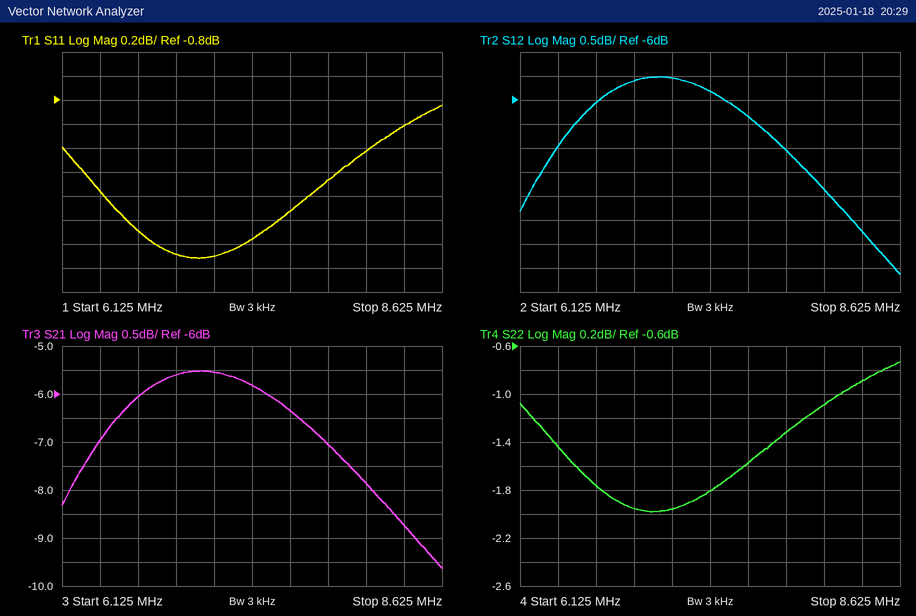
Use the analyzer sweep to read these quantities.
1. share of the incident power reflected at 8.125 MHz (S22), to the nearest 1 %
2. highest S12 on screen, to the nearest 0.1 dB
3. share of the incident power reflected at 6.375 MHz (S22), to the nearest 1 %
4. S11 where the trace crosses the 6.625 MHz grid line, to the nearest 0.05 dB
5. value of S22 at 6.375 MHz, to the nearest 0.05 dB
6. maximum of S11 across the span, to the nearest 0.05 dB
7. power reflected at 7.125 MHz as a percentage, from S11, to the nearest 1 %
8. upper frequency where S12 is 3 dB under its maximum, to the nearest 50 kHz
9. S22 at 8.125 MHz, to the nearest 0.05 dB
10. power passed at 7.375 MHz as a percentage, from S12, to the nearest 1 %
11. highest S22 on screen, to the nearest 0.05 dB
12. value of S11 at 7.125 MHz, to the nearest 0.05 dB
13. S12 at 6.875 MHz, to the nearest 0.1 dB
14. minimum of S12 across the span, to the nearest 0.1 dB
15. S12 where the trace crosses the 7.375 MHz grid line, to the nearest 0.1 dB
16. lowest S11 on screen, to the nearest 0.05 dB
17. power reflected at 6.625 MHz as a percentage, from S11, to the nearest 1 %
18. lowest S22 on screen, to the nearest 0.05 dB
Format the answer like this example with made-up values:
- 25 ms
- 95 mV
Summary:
- 78 %
- -5.5 dB
- 72 %
- -1.90 dB
- -1.45 dB
- -0.85 dB
- 62 %
- 8.30 MHz
- -1.10 dB
- 26 %
- -0.75 dB
- -2.10 dB
- -5.6 dB
- -9.6 dB
- -5.8 dB
- -2.10 dB
- 65 %
- -2.00 dB
